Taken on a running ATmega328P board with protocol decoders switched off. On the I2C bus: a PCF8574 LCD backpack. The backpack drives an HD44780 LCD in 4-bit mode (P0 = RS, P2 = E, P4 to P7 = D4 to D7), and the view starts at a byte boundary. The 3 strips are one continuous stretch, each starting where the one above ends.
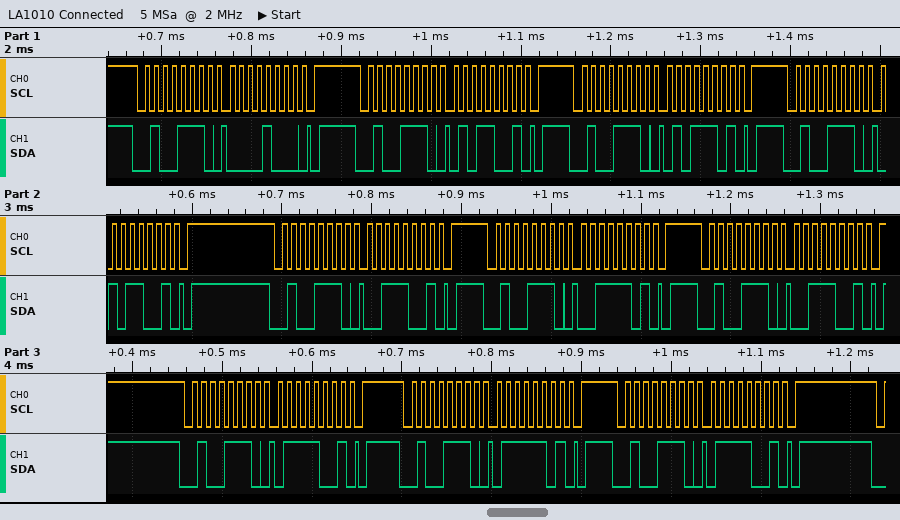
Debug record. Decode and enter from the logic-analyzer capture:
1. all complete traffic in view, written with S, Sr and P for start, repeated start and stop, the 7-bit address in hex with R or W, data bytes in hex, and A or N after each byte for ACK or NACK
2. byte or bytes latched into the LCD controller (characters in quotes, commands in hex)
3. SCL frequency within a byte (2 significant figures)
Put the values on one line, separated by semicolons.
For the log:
S 27W A 08 A P S 27W A 59 A P S 27W A 5D A P S 27W A 59 A P S 27W A 39 A P S 27W A 3D A P S 27W A 39 A P S 27W A 79 A P S 27W A 7D A P S 27W A 79 A P; 'S'; 100 kHz
